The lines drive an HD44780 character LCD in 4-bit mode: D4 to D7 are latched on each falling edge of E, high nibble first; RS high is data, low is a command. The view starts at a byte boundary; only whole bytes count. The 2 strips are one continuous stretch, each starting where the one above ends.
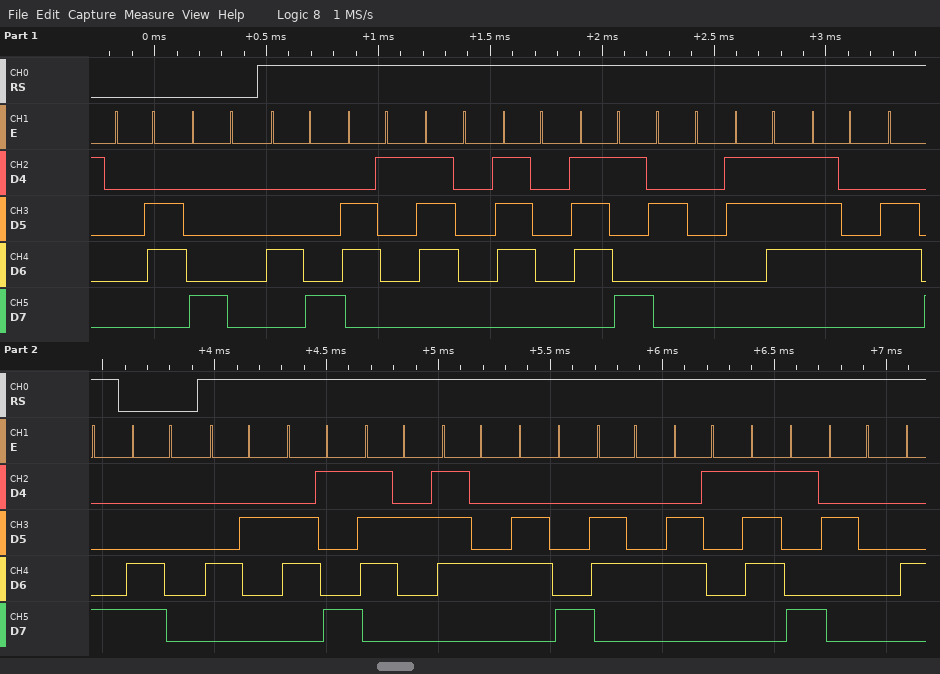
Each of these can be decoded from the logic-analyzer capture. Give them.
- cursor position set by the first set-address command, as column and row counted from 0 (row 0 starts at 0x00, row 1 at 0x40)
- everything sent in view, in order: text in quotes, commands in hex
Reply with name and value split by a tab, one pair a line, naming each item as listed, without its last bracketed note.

cursor position set by the first set-address command, as column and row counted from 0	column 0, row 0
everything sent in view, in order: text in quotes, commands in hex	0x06 0x80 "Happy 7th" 0xC0 "Birthday "
